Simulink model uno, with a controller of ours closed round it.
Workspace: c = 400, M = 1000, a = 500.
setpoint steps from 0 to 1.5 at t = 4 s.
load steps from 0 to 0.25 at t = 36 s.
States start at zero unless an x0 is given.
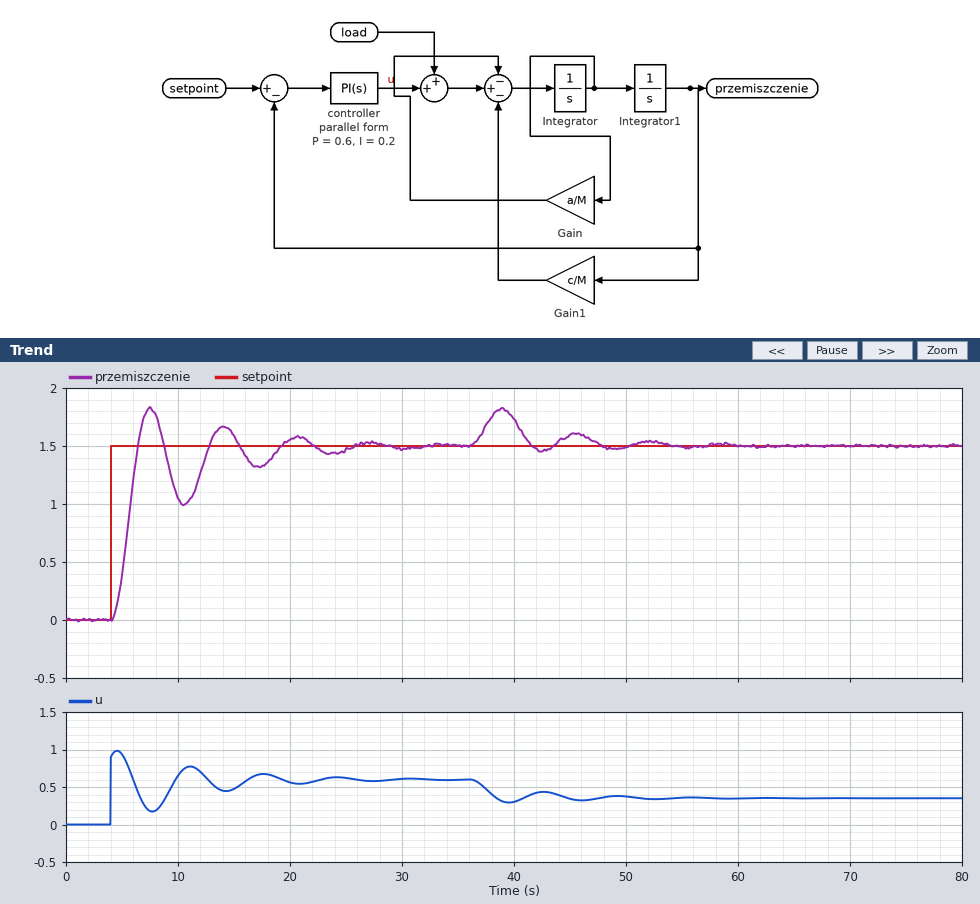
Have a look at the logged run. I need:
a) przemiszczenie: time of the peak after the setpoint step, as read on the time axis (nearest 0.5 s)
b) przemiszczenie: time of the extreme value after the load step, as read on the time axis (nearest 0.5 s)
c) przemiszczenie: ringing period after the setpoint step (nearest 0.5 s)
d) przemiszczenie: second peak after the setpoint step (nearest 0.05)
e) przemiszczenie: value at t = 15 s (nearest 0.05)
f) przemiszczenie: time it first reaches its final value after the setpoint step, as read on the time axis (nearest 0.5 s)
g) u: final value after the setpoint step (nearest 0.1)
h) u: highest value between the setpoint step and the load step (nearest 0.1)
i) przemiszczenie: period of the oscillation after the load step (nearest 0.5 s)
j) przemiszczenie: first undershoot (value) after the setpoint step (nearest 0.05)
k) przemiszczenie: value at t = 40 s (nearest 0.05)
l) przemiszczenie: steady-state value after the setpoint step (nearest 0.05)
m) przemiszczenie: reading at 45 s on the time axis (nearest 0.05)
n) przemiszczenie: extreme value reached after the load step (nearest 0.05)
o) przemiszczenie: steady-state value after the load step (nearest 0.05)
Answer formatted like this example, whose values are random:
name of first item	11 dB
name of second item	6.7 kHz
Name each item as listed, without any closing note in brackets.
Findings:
przemiszczenie: time of the peak after the setpoint step, as read on the time axis	7.5 s
przemiszczenie: time of the extreme value after the load step, as read on the time axis	39.0 s
przemiszczenie: ringing period after the setpoint step	6.5 s
przemiszczenie: second peak after the setpoint step	1.65
przemiszczenie: value at t = 15 s	1.60
przemiszczenie: time it first reaches its final value after the setpoint step, as read on the time axis	6.5 s
u: final value after the setpoint step	0.6
u: highest value between the setpoint step and the load step	1.0
przemiszczenie: period of the oscillation after the load step	6.5 s
przemiszczenie: first undershoot (value) after the setpoint step	1.00
przemiszczenie: value at t = 40 s	1.75
przemiszczenie: steady-state value after the setpoint step	1.50
przemiszczenie: reading at 45 s on the time axis	1.60
przemiszczenie: extreme value reached after the load step	1.80
przemiszczenie: steady-state value after the load step	1.50
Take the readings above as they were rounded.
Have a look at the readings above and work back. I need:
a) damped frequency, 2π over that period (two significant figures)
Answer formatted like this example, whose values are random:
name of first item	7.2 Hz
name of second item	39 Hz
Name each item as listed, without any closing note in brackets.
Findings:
damped frequency, 2π over that period	0.97 rad/s
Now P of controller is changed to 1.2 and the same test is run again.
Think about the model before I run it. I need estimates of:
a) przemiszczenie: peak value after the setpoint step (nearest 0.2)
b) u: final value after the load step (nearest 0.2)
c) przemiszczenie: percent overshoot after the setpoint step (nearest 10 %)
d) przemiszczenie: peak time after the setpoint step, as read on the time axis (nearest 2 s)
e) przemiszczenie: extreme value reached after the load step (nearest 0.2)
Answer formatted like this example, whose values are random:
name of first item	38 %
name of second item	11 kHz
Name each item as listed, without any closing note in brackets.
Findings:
przemiszczenie: peak value after the setpoint step	2.0
u: final value after the load step	0.4
przemiszczenie: percent overshoot after the setpoint step	30 %
przemiszczenie: peak time after the setpoint step, as read on the time axis	6 s
przemiszczenie: extreme value reached after the load step	1.8
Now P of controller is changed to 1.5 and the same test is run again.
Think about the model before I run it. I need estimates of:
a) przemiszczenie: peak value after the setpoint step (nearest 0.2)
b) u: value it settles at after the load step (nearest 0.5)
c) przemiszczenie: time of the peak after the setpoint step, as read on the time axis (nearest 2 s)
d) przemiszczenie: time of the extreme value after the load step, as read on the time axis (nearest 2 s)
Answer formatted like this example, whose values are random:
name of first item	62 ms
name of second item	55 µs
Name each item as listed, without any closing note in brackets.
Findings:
przemiszczenie: peak value after the setpoint step	2.0
u: value it settles at after the load step	0.5
przemiszczenie: time of the peak after the setpoint step, as read on the time axis	6 s
przemiszczenie: time of the extreme value after the load step, as read on the time axis	38 s
